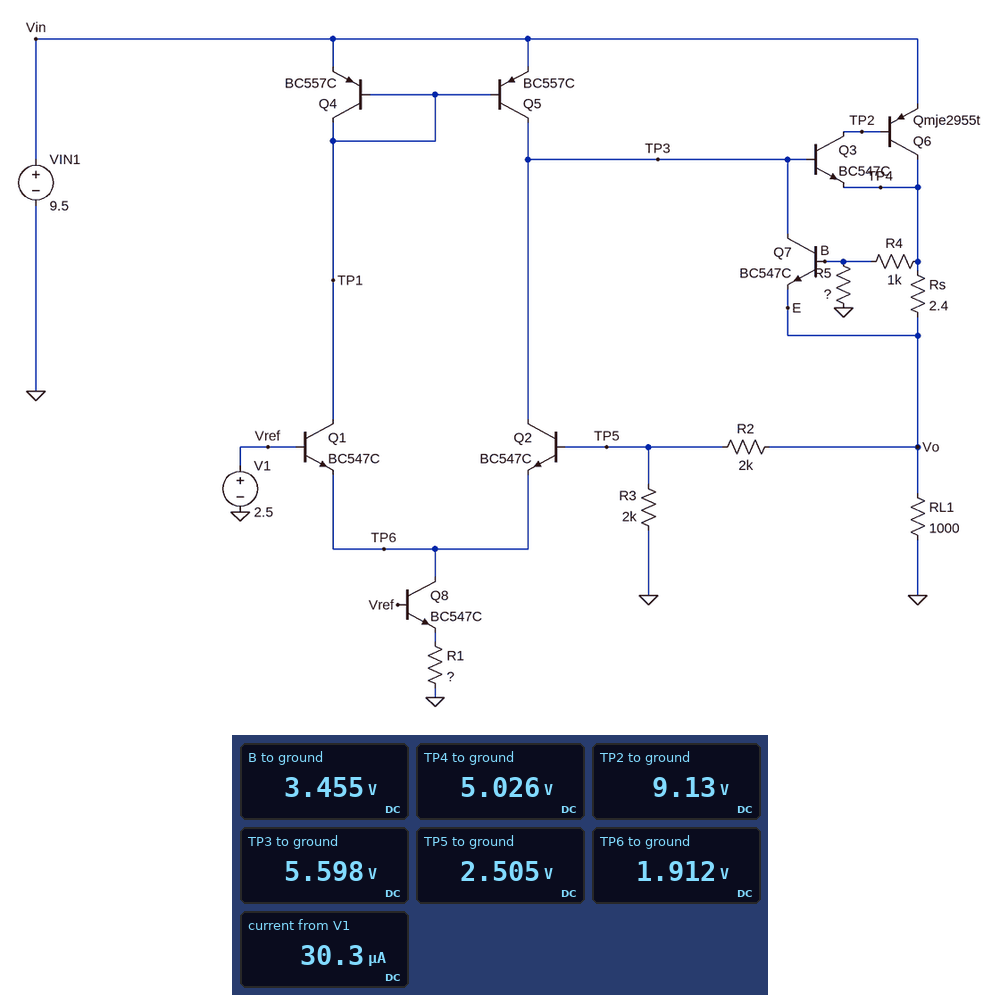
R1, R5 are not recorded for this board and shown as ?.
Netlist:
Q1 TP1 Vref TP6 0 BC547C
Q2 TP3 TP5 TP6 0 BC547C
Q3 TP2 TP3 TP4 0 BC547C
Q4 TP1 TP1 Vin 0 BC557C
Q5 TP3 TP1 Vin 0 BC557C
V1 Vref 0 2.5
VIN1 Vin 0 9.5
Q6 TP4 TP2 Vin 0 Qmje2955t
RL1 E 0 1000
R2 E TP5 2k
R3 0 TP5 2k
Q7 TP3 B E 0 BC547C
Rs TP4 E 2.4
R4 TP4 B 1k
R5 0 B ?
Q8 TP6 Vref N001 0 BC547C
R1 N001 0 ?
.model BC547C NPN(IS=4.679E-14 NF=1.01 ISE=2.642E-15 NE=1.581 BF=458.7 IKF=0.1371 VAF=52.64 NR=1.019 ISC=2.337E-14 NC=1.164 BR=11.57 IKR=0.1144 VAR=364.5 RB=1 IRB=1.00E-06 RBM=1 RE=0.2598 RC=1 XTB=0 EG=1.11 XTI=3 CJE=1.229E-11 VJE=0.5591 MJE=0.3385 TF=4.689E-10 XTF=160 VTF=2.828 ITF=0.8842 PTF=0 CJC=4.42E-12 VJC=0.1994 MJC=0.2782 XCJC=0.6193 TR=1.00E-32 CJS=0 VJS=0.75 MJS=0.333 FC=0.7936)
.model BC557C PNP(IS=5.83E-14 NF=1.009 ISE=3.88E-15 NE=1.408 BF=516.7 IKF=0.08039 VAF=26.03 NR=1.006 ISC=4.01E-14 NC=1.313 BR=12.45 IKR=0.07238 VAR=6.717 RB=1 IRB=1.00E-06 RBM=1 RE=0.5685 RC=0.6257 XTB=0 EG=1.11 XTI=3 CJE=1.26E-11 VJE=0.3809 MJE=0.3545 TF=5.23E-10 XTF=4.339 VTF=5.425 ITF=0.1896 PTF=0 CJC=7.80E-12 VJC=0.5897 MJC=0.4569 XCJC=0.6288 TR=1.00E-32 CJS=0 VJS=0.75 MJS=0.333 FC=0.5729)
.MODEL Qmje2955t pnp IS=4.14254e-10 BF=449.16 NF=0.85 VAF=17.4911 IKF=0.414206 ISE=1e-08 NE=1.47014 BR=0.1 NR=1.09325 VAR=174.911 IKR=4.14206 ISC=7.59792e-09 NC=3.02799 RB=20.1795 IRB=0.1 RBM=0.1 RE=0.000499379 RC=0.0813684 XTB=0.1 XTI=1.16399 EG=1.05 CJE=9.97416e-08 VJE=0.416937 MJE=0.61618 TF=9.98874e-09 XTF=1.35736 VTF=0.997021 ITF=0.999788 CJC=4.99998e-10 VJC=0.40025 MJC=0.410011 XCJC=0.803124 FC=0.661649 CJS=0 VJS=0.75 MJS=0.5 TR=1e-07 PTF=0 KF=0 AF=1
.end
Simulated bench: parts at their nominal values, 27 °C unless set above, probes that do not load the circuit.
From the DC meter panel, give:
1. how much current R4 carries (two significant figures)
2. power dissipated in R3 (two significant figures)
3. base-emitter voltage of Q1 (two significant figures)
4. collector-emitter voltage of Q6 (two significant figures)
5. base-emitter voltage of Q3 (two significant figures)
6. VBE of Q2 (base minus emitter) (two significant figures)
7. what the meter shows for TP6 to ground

1.6 mA
3.1 mW
590 mV
-4.5 V
570 mV
590 mV
1.912 V
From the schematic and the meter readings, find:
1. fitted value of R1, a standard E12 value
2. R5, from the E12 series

2.7 kΩ
2.2 kΩ
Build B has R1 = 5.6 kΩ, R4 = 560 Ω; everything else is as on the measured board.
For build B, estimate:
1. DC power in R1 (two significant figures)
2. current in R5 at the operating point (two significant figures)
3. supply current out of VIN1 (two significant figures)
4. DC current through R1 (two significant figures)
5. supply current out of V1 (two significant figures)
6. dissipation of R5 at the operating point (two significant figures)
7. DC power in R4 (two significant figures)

640 µW
1.8 mA
8.4 mA
340 µA
15 µA
7.3 mW
1.9 mW
